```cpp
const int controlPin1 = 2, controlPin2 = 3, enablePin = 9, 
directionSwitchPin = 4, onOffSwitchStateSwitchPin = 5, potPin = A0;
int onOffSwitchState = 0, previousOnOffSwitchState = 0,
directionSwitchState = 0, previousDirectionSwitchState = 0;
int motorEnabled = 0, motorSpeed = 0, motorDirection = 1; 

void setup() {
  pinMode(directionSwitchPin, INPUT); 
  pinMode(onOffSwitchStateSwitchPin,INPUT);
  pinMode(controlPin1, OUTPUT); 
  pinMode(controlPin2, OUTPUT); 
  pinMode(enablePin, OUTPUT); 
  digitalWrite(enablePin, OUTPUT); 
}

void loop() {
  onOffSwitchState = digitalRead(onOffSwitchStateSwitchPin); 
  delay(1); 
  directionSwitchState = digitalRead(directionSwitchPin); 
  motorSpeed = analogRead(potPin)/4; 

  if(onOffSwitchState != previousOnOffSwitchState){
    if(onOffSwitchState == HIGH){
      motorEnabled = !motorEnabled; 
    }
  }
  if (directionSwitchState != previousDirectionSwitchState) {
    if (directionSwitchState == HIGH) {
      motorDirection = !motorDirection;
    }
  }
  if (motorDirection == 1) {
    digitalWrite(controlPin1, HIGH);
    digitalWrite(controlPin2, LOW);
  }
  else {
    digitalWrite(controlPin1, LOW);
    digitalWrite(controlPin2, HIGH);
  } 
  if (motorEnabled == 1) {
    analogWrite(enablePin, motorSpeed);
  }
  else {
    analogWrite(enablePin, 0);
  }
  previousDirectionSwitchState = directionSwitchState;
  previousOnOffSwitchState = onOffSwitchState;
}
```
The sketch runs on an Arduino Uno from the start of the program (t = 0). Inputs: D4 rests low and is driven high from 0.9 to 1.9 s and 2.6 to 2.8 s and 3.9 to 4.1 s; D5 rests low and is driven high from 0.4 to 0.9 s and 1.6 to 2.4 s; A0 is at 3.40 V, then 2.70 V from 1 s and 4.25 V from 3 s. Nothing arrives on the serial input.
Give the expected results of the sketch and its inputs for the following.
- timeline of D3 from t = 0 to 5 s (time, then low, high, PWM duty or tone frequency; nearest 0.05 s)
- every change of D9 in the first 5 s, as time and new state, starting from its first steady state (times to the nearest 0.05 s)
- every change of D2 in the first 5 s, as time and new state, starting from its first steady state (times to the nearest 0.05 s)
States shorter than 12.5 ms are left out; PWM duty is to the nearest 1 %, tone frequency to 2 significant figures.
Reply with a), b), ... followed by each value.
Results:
a) 0 s low; 0.9 s high; 2.6 s low; 3.9 s high
b) 0 s low; 0.4 s PWM 68 %; 1 s PWM 54 %; 1.6 s low
c) 0 s high; 0.9 s low; 2.6 s high; 3.9 s low
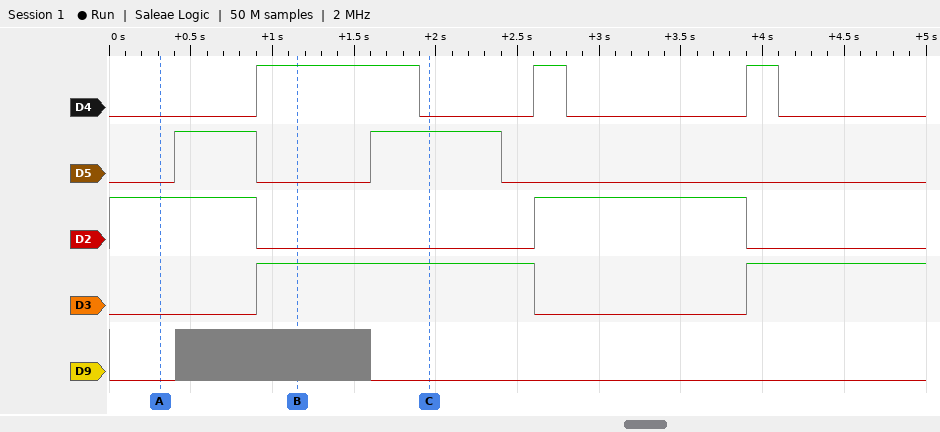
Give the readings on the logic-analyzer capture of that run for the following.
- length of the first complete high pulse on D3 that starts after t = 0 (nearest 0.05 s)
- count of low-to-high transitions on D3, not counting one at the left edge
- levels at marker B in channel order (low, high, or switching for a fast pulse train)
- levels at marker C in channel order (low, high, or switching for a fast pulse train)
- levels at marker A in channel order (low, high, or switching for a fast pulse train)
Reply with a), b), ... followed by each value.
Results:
a) 1.70 s
b) 2
c) D4 high, D5 low, D2 low, D3 high, D9 switching
d) D4 low, D5 high, D2 low, D3 high, D9 low
e) D4 low, D5 low, D2 high, D3 low, D9 low
